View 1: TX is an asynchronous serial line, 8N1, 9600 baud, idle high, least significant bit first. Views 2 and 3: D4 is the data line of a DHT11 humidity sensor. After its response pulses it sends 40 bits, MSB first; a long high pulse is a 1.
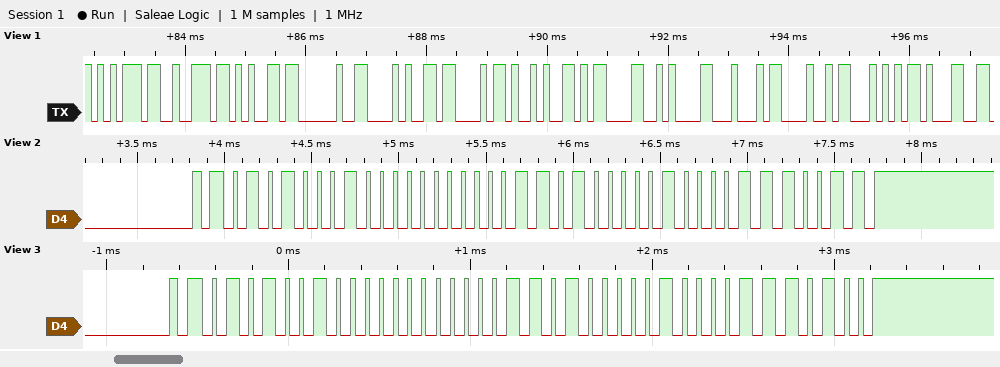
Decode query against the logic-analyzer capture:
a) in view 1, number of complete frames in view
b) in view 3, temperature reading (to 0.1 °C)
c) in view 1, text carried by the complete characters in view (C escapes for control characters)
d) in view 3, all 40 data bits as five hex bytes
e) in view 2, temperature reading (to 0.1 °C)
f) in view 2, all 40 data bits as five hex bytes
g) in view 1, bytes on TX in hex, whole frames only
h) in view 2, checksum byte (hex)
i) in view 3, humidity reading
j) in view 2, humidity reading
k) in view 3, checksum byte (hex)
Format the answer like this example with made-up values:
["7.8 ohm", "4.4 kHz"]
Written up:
["13", "26.8 °C", "\"ure (C)\\r\\nDHT1\"", "52 00 1A 08 74", "26.8 °C", "51 00 1A 08 73", "75 72 65 20 28 43 29 0D 0A 44 48 54 31", "0x73", "82 %", "81 %", "0x74"]
